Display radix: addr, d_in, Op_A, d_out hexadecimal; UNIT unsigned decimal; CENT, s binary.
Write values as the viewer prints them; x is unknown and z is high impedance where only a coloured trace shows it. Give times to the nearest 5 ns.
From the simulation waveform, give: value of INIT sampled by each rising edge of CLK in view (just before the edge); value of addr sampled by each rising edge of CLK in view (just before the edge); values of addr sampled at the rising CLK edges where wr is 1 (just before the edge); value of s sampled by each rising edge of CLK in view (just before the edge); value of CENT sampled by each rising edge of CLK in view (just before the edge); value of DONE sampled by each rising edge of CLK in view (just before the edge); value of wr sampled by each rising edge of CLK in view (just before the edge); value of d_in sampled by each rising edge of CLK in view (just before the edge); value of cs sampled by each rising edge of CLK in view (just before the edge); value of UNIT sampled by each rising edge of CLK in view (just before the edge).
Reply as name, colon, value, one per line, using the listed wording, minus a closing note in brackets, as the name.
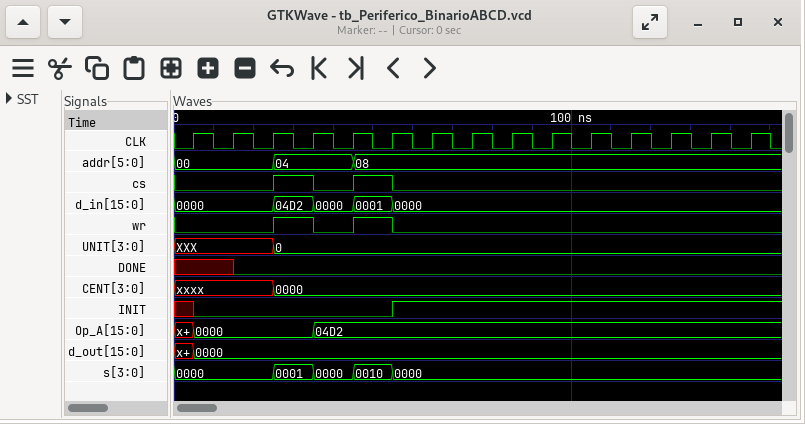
value of INIT sampled by each rising edge of CLK in view: x 0 0 0 0 0 1 1 1 1 1 1 1 1 1
value of addr sampled by each rising edge of CLK in view: 00, 00, 00, 04, 04, 08, 08, 08, 08, 08, 08, 08, 08, 08, 08
values of addr sampled at the rising CLK edges where wr is 1: 04, 08
value of s sampled by each rising edge of CLK in view: 0000, 0000, 0000, 0001, 0000, 0010, 0000, 0000, 0000, 0000, 0000, 0000, 0000, 0000, 0000
value of CENT sampled by each rising edge of CLK in view: xxxx, xxxx, xxxx, 0000, 0000, 0000, 0000, 0000, 0000, 0000, 0000, 0000, 0000, 0000, 0000
value of DONE sampled by each rising edge of CLK in view: x x 0 0 0 0 0 0 0 0 0 0 0 0 0
value of wr sampled by each rising edge of CLK in view: 0 0 0 1 0 1 0 0 0 0 0 0 0 0 0
value of d_in sampled by each rising edge of CLK in view: 0000, 0000, 0000, 04D2, 0000, 0001, 0000, 0000, 0000, 0000, 0000, 0000, 0000, 0000, 0000
value of cs sampled by each rising edge of CLK in view: 0 0 0 1 0 1 0 0 0 0 0 0 0 0 0
value of UNIT sampled by each rising edge of CLK in view: XXX, XXX, XXX, 0, 0, 0, 0, 0, 0, 0, 0, 0, 0, 0, 0
